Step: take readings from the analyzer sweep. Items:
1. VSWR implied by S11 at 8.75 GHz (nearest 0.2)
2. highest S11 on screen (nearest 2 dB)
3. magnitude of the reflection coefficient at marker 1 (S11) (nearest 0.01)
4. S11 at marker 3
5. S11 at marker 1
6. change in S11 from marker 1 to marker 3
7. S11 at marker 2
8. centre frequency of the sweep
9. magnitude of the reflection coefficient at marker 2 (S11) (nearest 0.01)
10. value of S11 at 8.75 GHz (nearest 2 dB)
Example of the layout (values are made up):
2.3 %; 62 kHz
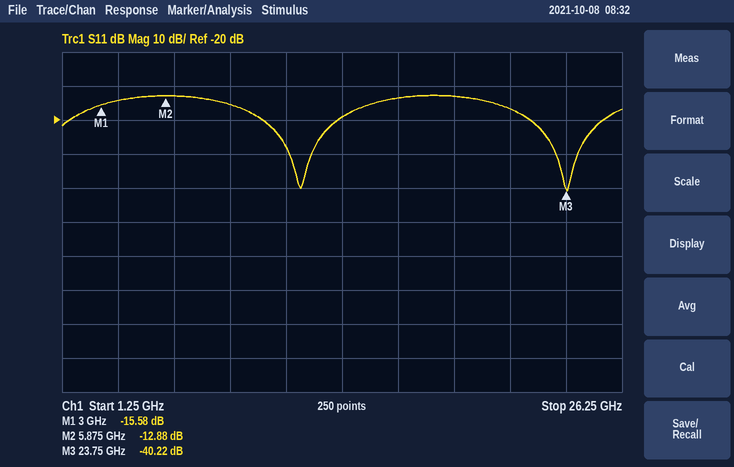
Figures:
1.4; -12 dB; 0.17; -40.22 dB; -15.58 dB; -24.64 dB; -12.88 dB; 13.75 GHz; 0.23; -16 dB
